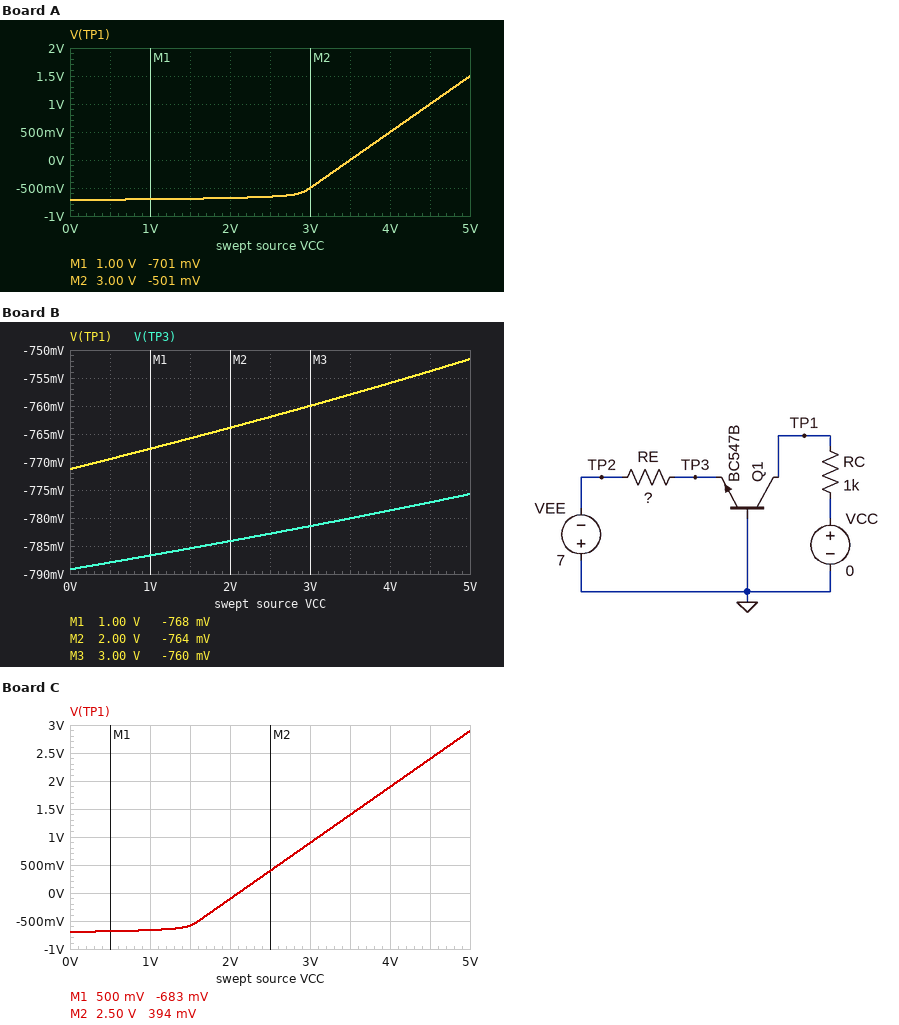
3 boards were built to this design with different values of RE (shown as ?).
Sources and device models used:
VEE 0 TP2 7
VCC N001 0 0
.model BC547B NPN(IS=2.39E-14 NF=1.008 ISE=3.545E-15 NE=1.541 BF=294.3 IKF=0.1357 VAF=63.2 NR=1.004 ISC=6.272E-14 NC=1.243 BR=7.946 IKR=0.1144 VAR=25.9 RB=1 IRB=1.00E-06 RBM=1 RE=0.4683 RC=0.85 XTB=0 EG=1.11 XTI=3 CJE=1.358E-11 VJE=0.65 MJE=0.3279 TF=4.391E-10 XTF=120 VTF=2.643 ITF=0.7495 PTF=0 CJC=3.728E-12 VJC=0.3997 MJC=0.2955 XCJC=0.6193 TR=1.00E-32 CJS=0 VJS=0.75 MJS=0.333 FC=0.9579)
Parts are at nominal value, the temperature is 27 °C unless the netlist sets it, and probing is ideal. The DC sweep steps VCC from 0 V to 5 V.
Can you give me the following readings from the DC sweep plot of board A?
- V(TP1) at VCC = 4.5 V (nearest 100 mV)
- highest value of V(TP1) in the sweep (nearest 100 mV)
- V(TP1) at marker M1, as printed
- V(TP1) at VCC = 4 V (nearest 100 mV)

1.0 V
1.5 V
-701 mV
500 mV
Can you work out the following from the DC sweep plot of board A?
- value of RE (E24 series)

1.8 kΩ
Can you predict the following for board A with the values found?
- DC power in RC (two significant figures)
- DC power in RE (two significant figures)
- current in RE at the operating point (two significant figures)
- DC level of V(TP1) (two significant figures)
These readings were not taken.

510 µW
22 mW
3.5 mA
-710 mV
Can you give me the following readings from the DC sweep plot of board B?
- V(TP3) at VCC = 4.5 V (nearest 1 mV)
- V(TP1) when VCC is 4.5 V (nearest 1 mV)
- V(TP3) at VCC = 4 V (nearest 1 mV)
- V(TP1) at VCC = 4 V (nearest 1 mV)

-777 mV
-754 mV
-779 mV
-756 mV
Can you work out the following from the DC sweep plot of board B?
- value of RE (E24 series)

390 Ω
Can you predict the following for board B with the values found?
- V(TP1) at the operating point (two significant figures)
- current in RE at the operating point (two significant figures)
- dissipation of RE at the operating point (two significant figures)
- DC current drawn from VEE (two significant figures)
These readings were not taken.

-770 mV
16 mA
99 mW
16 mA
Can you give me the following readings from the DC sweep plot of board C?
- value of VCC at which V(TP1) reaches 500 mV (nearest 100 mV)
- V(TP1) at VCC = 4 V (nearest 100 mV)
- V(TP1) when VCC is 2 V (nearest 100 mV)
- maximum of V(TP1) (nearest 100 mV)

2.6 V
1.9 V
-100 mV
2.9 V
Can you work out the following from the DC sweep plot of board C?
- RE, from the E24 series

3 kΩ
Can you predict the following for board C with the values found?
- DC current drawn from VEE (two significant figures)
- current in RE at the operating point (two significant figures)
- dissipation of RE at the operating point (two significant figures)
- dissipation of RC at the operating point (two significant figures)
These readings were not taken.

2.1 mA
2.1 mA
13 mW
480 µW
